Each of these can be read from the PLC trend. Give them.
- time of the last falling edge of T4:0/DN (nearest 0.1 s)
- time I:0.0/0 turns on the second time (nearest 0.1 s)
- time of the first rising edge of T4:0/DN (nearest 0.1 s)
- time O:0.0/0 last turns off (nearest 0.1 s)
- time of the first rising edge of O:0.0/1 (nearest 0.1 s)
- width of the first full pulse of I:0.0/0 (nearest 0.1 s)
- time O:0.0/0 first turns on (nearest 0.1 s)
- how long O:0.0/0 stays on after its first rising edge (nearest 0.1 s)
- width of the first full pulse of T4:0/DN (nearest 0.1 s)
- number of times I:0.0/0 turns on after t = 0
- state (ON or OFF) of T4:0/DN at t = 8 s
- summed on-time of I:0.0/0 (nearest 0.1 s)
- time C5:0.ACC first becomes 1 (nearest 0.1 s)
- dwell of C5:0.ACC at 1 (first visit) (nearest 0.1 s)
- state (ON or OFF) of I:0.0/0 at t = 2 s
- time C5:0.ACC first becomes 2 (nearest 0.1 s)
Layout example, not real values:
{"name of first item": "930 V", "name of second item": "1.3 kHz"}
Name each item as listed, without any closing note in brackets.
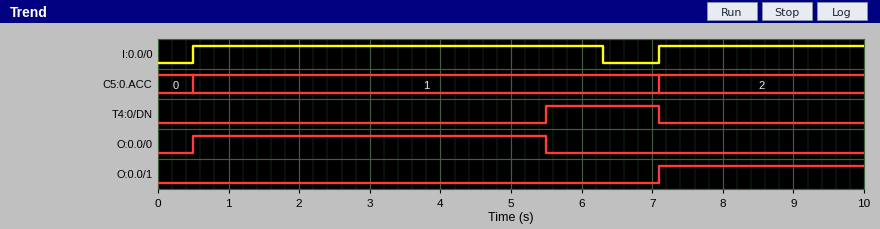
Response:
{"time of the last falling edge of T4:0/DN": "7.1 s", "time I:0.0/0 turns on the second time": "7.1 s", "time of the first rising edge of T4:0/DN": "5.5 s", "time O:0.0/0 last turns off": "5.5 s", "time of the first rising edge of O:0.0/1": "7.1 s", "width of the first full pulse of I:0.0/0": "5.8 s", "time O:0.0/0 first turns on": "0.5 s", "how long O:0.0/0 stays on after its first rising edge": "5.0 s", "width of the first full pulse of T4:0/DN": "1.6 s", "number of times I:0.0/0 turns on after t = 0": "2", "state (ON or OFF) of T4:0/DN at t = 8 s": "OFF", "summed on-time of I:0.0/0": "8.7 s", "time C5:0.ACC first becomes 1": "0.5 s", "dwell of C5:0.ACC at 1 (first visit)": "6.6 s", "state (ON or OFF) of I:0.0/0 at t = 2 s": "ON", "time C5:0.ACC first becomes 2": "7.1 s"}
